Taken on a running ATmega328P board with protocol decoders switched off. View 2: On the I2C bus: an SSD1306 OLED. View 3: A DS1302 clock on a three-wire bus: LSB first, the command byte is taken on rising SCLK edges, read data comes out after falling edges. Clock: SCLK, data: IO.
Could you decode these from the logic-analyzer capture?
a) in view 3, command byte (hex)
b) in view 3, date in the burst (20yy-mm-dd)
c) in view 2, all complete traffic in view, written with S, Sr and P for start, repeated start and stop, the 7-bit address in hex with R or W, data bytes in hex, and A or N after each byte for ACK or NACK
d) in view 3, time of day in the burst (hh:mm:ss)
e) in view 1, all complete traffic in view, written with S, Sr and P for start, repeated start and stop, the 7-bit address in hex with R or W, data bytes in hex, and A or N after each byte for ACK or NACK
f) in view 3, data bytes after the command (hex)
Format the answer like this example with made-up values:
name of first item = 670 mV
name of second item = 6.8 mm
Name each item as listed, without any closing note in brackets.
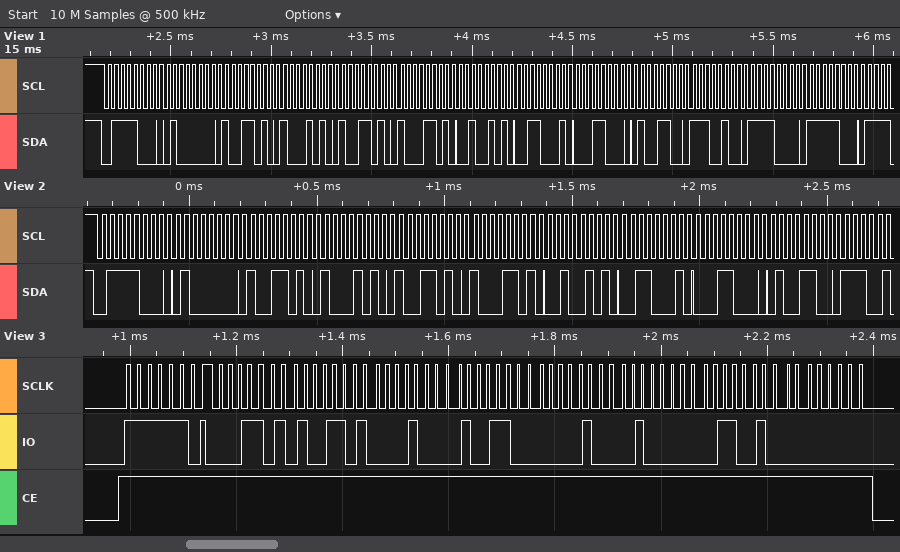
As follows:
in view 3, command byte = 0xBF
in view 3, date in the burst = 2026-10-19
in view 2, all complete traffic in view, written with S, Sr and P for start, repeated start and stop, the 7-bit address in hex with R or W, data bytes in hex, and A or N after each byte for ACK or NACK = S 3CW A 40 A 9A A 8A A 9A A 8D A 25 A 31 A 18 A 4C A
in view 3, time of day in the burst = 08:59:58
in view 1, all complete traffic in view, written with S, Sr and P for start, repeated start and stop, the 7-bit address in hex with R or W, data bytes in hex, and A or N after each byte for ACK or NACK = S 3CW A 40 A 9A A 8A A 9A A 8D A 25 A 31 A 18 A 4C A E4 A F0 A F8 A
in view 3, data bytes after the command = 58 59 08 19 10 02 26 00
